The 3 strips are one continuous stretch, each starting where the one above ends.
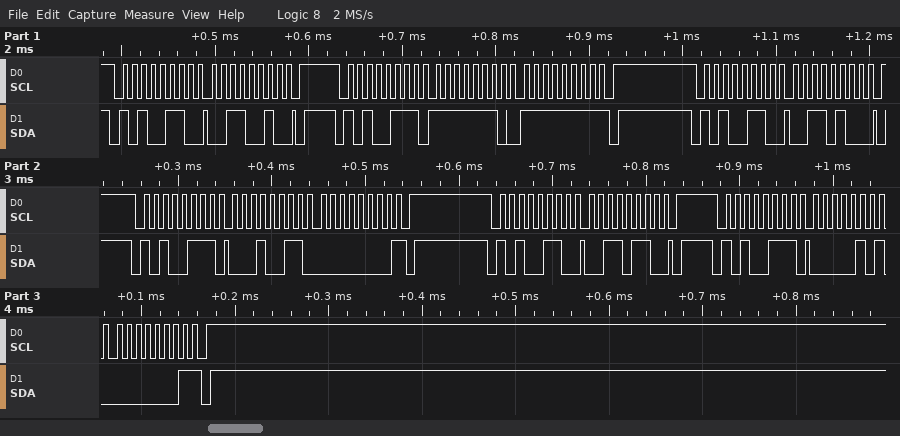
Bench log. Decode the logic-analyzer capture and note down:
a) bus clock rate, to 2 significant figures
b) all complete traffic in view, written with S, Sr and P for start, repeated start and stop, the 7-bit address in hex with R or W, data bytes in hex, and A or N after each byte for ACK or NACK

100 kHz
S 53W A 32 A P S 53R A FE A FF N P S 53W A 34 A P S 53R A 13 A 00 N P S 53W A 36 A P S 53R A 05 A 01 N P
